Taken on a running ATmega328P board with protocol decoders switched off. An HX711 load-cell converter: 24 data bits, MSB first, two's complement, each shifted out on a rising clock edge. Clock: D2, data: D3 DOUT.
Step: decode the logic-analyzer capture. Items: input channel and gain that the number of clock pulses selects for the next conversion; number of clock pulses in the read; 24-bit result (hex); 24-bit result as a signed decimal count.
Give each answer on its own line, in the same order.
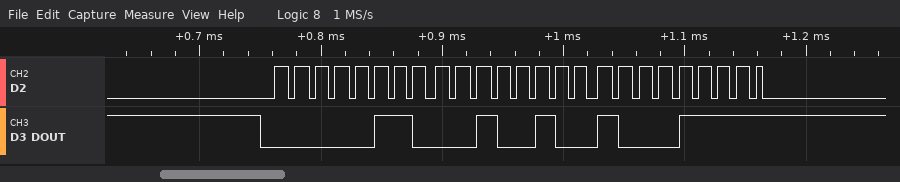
channel A, gain 128
25
0x06248F
402575
